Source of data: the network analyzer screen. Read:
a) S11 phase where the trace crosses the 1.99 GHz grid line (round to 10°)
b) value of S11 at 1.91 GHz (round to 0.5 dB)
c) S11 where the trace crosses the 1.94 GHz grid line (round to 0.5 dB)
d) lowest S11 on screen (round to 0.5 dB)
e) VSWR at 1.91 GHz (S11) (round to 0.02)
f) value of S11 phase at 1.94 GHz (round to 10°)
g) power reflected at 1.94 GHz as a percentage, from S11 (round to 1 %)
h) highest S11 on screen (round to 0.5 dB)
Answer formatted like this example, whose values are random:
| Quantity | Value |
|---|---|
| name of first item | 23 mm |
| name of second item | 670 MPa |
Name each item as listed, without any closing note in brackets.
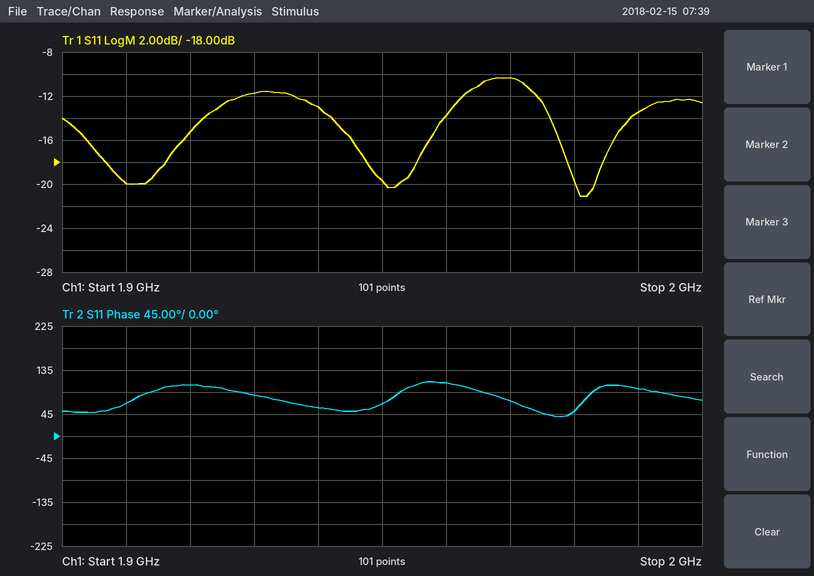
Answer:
| Quantity | Value |
|---|---|
| S11 phase where the trace crosses the 1.99 GHz grid line | 100° |
| value of S11 at 1.91 GHz | -20.0 dB |
| S11 where the trace crosses the 1.94 GHz grid line | -13.0 dB |
| lowest S11 on screen | -21.0 dB |
| VSWR at 1.91 GHz (S11) | 1.22 |
| value of S11 phase at 1.94 GHz | 60° |
| power reflected at 1.94 GHz as a percentage, from S11 | 5 % |
| highest S11 on screen | -10.5 dB |
